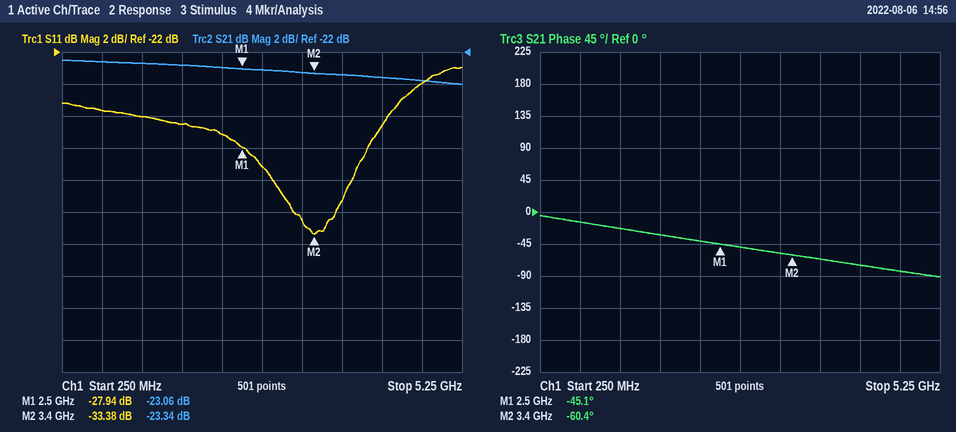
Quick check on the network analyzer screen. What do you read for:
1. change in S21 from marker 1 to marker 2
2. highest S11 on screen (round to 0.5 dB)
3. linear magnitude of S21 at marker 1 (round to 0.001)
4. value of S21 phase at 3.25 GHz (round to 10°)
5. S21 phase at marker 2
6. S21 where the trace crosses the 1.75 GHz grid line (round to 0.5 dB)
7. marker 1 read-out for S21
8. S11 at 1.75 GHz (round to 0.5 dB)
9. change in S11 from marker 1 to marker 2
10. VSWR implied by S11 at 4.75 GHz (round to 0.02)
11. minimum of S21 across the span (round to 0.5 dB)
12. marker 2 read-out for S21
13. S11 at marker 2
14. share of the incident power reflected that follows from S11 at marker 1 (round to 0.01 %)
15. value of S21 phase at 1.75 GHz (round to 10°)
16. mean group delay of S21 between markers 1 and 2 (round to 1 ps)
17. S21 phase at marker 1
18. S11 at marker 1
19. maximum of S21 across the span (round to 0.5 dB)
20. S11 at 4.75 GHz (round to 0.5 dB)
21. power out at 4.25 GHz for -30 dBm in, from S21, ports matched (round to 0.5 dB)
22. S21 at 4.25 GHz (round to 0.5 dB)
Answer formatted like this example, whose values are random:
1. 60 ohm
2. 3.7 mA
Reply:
1. -0.28 dB
2. -23.0 dB
3. 0.070
4. -60°
5. -60.4°
6. -23.0 dB
7. -23.06 dB
8. -26.5 dB
9. -5.44 dB
10. 1.14
11. -24.0 dB
12. -23.34 dB
13. -33.38 dB
14. 0.16 %
15. -30°
16. 47 ps
17. -45.1°
18. -27.94 dB
19. -22.5 dB
20. -24.0 dB
21. -53.5 dBm
22. -23.5 dB
